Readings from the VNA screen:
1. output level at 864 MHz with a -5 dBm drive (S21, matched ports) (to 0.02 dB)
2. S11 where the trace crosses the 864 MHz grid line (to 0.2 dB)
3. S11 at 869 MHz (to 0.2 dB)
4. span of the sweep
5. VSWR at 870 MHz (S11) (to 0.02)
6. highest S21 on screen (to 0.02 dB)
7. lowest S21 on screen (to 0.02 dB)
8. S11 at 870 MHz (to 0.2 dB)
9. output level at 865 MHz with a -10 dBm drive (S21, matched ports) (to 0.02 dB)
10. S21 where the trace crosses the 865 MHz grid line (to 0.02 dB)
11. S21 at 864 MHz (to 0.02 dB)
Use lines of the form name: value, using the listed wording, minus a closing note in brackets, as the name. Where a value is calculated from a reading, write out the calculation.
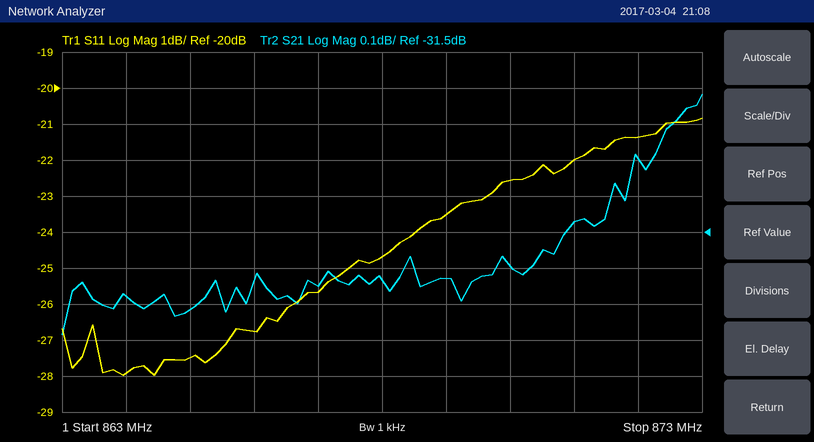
output level at 864 MHz with a -5 dBm drive (S21, matched ports): -5 dBm + (-31.68 dB) = -36.68 dBm
S11 where the trace crosses the 864 MHz grid line: -28.0 dB
S11 at 869 MHz: -23.6 dB
span of the sweep: 10 MHz
VSWR at 870 MHz (S11): |Γ| = 10^(-22.6/20) = 0.0741; VSWR = (1 + 0.0741)/(1 − 0.0741) ≈ 1.16
highest S21 on screen: -31.12 dB
lowest S21 on screen: -31.78 dB
S11 at 870 MHz: -22.6 dB
output level at 865 MHz with a -10 dBm drive (S21, matched ports): -10 dBm + (-31.72 dB) = -41.72 dBm
S21 where the trace crosses the 865 MHz grid line: -31.72 dB
S21 at 864 MHz: -31.68 dB
